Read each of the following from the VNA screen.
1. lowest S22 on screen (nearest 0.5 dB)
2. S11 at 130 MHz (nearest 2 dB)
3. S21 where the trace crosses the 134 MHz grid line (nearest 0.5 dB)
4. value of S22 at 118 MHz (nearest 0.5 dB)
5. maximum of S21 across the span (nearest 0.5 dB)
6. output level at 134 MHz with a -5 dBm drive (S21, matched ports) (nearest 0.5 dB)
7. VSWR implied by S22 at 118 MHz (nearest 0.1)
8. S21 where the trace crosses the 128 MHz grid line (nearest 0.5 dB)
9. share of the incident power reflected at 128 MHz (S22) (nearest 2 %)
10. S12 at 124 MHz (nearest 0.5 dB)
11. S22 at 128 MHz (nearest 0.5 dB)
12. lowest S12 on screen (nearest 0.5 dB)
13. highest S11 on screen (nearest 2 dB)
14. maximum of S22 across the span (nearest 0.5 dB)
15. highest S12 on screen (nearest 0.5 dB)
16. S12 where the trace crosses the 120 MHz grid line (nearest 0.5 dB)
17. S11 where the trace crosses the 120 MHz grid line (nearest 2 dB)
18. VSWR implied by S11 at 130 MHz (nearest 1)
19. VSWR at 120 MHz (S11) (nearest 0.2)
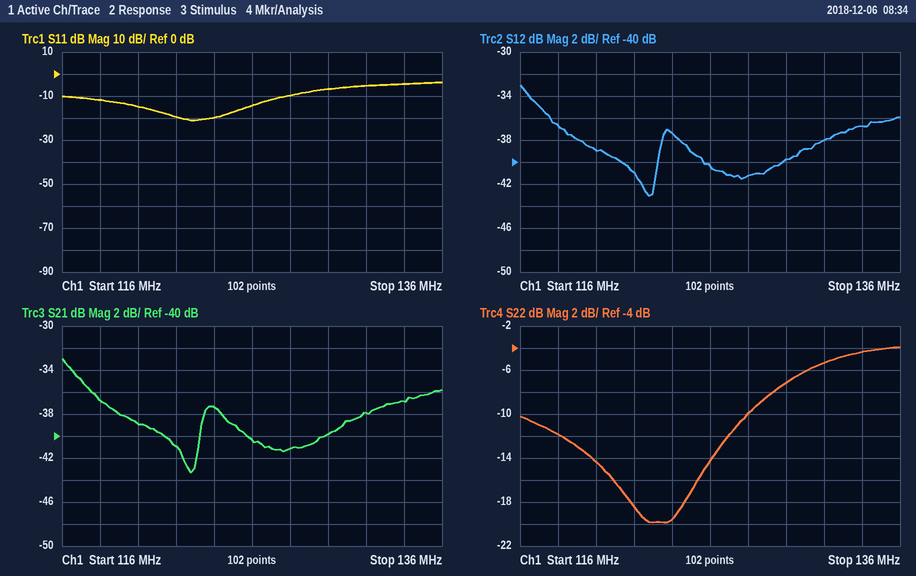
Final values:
-20.0 dB
-6 dB
-37.0 dB
-12.0 dB
-33.0 dB
-42.0 dBm
1.7
-41.0 dB
10 %
-37.5 dB
-10.0 dB
-43.0 dB
-4 dB
-4.0 dB
-33.0 dB
-39.0 dB
-14 dB
3
1.4
